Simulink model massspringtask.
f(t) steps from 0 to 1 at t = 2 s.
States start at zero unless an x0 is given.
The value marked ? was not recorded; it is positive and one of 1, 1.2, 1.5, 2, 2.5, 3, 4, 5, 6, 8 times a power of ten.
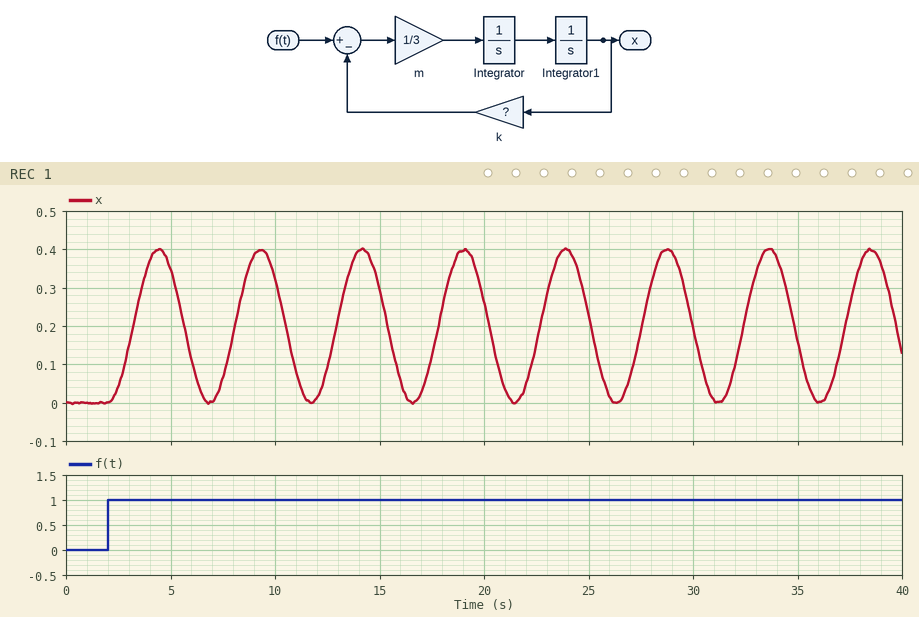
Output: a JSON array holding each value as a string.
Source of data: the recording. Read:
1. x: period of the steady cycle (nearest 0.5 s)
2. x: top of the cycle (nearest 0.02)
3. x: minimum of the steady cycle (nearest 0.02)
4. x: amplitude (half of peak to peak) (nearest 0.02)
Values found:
["5.0 s", "0.40", "0.00", "0.20"]
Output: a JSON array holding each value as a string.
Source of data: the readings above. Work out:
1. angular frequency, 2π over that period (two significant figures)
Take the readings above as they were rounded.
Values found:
["1.3 rad/s"]
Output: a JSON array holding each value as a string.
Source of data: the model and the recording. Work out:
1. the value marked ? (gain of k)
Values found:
["5"]
